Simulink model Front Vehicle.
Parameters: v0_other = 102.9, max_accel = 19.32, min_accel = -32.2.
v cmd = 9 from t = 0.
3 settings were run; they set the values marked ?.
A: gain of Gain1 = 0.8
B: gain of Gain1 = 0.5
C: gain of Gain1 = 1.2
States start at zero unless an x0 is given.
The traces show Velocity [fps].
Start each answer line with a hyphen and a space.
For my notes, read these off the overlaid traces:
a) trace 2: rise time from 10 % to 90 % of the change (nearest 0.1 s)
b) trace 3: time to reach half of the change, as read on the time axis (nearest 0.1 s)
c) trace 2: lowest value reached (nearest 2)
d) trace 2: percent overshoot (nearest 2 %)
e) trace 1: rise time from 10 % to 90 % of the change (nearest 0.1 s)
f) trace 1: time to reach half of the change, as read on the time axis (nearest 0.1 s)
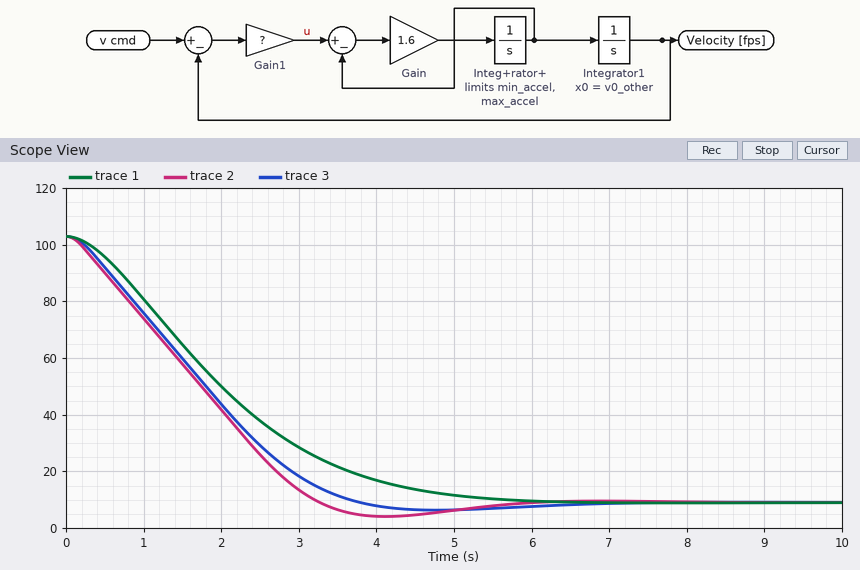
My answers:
- 2.4 s
- 1.6 s
- 4
- 6 %
- 3.2 s
- 1.8 s
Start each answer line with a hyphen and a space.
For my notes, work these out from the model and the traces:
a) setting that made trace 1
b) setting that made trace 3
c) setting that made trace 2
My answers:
- B
- A
- C
